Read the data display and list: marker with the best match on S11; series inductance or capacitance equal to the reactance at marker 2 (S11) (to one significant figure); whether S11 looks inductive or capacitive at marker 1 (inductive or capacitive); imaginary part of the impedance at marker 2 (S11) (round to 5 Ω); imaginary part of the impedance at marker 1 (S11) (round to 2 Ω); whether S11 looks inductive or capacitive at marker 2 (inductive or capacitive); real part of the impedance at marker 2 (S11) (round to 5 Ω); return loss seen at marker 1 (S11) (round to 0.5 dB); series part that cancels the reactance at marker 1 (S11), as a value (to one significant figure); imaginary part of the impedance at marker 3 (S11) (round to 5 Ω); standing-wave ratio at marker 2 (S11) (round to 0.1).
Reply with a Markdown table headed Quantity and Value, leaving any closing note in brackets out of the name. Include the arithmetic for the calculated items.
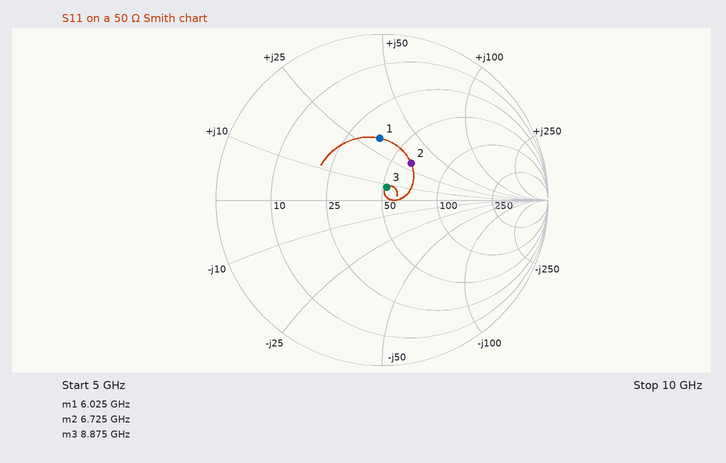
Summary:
| Quantity | Value |
|---|---|
| marker with the best match on S11 | marker 3 |
| series inductance or capacitance equal to the reactance at marker 2 (S11) | L = 30 Ω/(2π × 6.725 GHz) ≈ 710 pH, so 700 pH to one significant figure |
| whether S11 looks inductive or capacitive at marker 1 | inductive |
| imaginary part of the impedance at marker 2 (S11) | +30 Ω |
| imaginary part of the impedance at marker 1 (S11) | +32 Ω |
| whether S11 looks inductive or capacitive at marker 2 | inductive |
| real part of the impedance at marker 2 (S11) | 65 Ω |
| return loss seen at marker 1 (S11) | 8.5 dB |
| series part that cancels the reactance at marker 1 (S11), as a value | C = 1/(2π × 6.025 GHz × 32 Ω) ≈ 825 fF, so 800 fF to one significant figure |
| imaginary part of the impedance at marker 3 (S11) | +10 Ω |
| standing-wave ratio at marker 2 (S11) | 1.8 |
